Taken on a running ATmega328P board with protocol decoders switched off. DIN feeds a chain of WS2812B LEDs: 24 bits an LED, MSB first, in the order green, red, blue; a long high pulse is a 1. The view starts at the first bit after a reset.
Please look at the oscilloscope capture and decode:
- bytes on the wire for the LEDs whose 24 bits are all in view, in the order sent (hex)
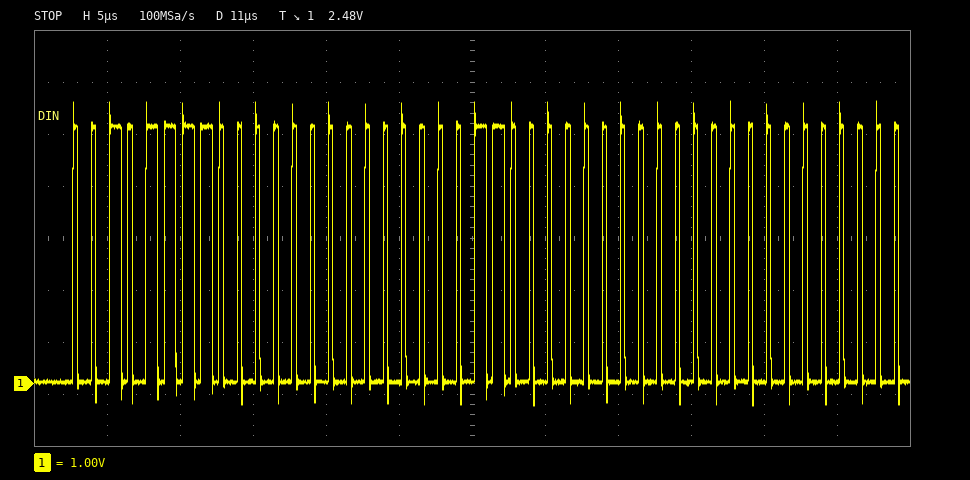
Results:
2F 00 03
